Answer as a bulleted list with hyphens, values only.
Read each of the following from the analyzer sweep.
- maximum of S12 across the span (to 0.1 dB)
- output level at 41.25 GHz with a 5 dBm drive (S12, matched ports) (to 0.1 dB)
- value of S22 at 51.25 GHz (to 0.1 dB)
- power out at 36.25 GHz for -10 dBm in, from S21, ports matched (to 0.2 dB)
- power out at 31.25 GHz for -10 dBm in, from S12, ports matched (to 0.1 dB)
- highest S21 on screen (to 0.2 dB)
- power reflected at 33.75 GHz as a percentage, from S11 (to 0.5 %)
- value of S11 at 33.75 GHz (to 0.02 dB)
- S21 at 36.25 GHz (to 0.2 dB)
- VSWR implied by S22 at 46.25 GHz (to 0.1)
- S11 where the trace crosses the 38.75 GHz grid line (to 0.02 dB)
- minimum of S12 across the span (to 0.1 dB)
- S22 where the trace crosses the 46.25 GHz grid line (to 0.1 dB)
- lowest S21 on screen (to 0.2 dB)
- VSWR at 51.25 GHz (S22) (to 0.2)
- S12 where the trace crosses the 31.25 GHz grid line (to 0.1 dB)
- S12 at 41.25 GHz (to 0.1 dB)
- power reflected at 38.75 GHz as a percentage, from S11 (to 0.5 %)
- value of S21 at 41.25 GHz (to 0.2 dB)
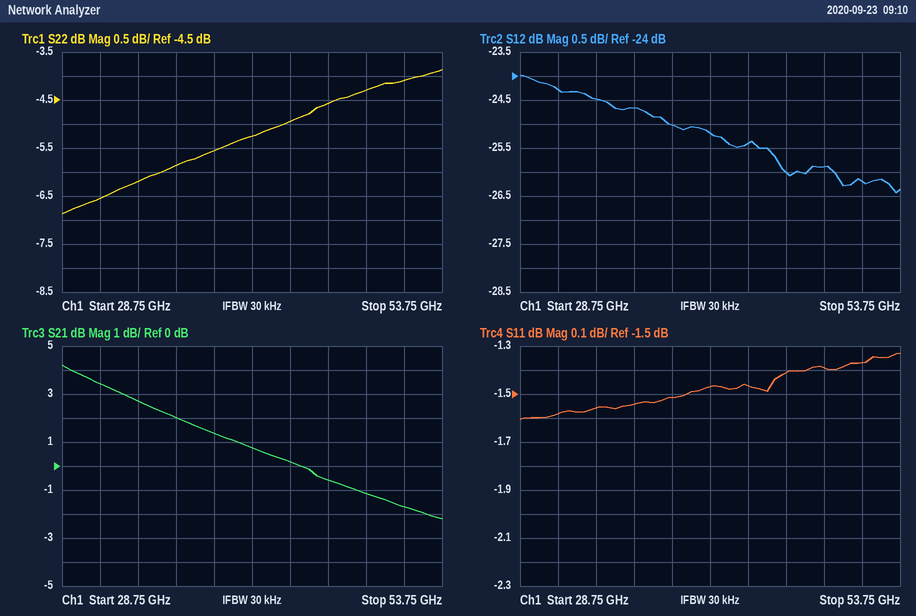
- -24.0 dB
- -20.2 dBm
- -4.1 dB
- -8.0 dBm
- -34.3 dBm
- 4.2 dB
- 70.0 %
- -1.56 dB
- 2.0 dB
- 3.9
- -1.52 dB
- -26.4 dB
- -4.6 dB
- -2.2 dB
- 4.4
- -24.3 dB
- -25.2 dB
- 70.5 %
- 0.8 dB
